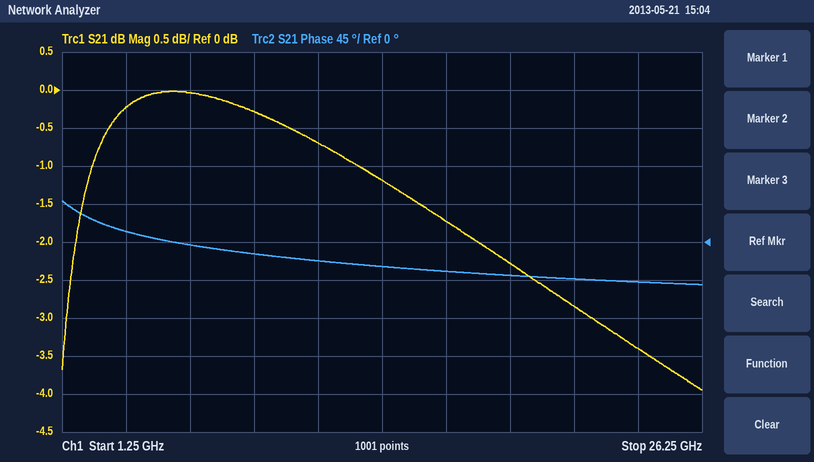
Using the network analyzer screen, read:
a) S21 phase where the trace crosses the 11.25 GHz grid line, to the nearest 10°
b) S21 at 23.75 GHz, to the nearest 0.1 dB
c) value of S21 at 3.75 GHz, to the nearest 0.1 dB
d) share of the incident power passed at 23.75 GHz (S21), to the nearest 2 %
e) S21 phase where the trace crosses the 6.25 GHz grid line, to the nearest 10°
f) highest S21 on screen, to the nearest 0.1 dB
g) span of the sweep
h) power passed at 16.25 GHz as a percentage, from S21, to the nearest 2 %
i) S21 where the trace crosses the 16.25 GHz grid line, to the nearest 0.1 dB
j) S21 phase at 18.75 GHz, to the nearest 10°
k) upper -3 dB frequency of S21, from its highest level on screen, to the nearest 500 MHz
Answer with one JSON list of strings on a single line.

["-20°", "-3.4 dB", "-0.2 dB", "46 %", "0°", "0.0 dB", "25 GHz", "68 %", "-1.7 dB", "-40°", "22.0 GHz"]
